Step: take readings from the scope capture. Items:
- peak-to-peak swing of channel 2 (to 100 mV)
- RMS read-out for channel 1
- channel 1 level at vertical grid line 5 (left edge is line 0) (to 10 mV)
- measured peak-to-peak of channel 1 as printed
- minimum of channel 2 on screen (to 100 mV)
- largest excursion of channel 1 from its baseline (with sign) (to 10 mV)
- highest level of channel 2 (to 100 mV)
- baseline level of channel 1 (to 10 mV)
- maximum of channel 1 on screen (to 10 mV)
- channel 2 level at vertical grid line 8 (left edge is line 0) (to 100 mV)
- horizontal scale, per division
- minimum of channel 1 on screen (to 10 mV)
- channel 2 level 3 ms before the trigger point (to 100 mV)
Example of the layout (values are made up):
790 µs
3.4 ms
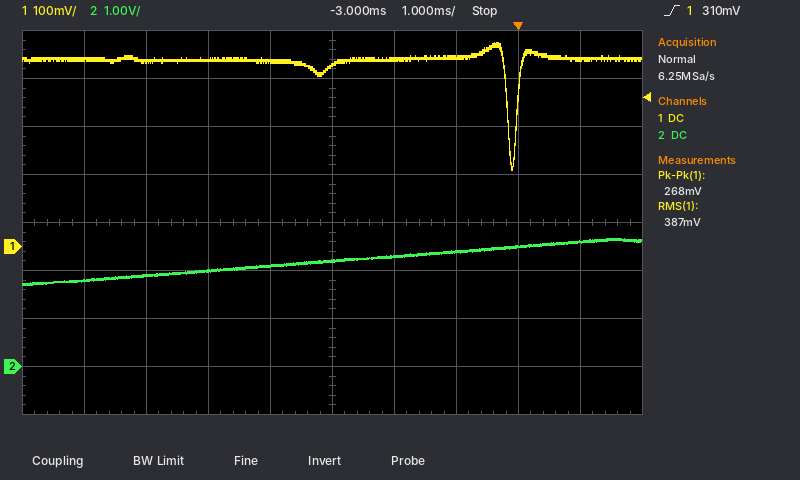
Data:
1.0 V
387 mV
380 mV
268 mV
1.7 V
-230 mV
2.7 V
390 mV
430 mV
2.5 V
1 ms
160 mV
2.2 V
